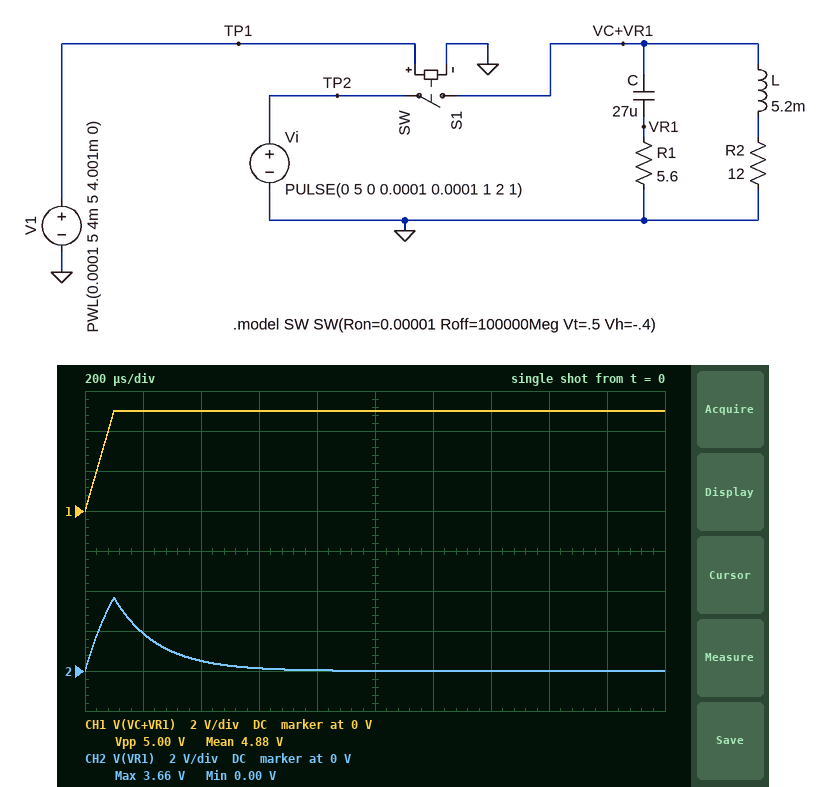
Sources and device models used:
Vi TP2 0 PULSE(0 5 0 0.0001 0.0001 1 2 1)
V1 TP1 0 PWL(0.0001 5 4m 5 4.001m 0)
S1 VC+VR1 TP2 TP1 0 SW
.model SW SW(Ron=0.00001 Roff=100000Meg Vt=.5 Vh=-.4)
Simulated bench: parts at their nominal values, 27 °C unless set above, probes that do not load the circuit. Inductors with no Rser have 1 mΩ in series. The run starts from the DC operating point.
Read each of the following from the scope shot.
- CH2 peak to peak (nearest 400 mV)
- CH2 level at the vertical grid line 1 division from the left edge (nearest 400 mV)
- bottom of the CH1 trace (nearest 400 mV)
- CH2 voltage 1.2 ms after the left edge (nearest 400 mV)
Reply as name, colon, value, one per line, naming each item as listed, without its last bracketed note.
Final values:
CH2 peak to peak: 3.6 V
CH2 level at the vertical grid line 1 division from the left edge: 2.0 V
bottom of the CH1 trace: 0 V
CH2 voltage 1.2 ms after the left edge: 0 V
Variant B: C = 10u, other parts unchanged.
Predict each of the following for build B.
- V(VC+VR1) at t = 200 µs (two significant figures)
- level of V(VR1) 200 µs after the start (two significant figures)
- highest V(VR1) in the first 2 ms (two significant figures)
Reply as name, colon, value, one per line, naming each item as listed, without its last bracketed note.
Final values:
V(VC+VR1) at t = 200 µs: 5.0 V
level of V(VR1) 200 µs after the start: 390 mV
highest V(VR1) in the first 2 ms: 2.3 V
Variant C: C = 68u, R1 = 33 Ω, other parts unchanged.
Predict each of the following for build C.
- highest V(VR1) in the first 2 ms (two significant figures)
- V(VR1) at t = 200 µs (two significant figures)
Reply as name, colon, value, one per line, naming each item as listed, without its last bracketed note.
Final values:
highest V(VR1) in the first 2 ms: 4.9 V
V(VR1) at t = 200 µs: 4.7 V
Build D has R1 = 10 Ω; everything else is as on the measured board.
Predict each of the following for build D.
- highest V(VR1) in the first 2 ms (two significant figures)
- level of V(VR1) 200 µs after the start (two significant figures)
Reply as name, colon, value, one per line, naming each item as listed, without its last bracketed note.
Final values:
highest V(VR1) in the first 2 ms: 4.2 V
level of V(VR1) 200 µs after the start: 2.9 V
